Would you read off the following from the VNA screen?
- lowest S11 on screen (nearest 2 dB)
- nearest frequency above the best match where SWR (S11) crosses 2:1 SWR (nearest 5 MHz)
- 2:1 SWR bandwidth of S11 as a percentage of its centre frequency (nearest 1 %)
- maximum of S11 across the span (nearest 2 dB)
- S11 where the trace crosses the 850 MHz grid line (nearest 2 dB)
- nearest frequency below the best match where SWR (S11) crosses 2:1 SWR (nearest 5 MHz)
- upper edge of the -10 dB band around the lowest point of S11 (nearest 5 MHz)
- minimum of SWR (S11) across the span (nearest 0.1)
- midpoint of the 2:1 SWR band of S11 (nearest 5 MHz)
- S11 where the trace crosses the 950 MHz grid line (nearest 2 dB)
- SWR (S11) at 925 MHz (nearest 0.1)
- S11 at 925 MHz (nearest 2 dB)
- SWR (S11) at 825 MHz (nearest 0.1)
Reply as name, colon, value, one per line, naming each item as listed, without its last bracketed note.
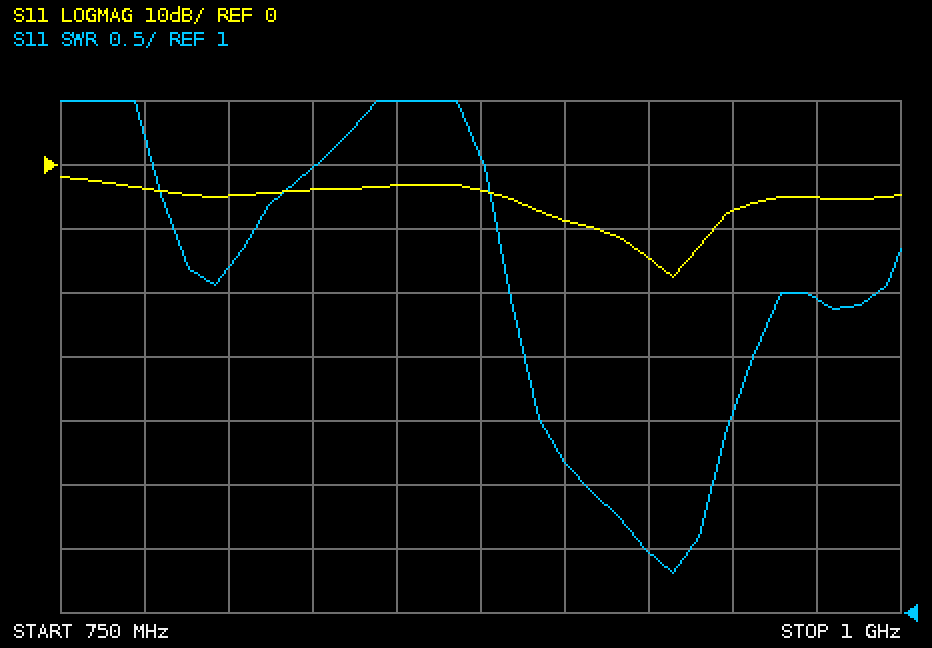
lowest S11 on screen: -18 dB
nearest frequency above the best match where SWR (S11) crosses 2:1 SWR: 945 MHz
2:1 SWR bandwidth of S11 as a percentage of its centre frequency: 4 %
maximum of S11 across the span: -2 dB
S11 where the trace crosses the 850 MHz grid line: -4 dB
nearest frequency below the best match where SWR (S11) crosses 2:1 SWR: 905 MHz
upper edge of the -10 dB band around the lowest point of S11: 945 MHz
minimum of SWR (S11) across the span: 1.3
midpoint of the 2:1 SWR band of S11: 925 MHz
S11 where the trace crosses the 950 MHz grid line: -8 dB
SWR (S11) at 925 MHz: 1.5
S11 at 925 MHz: -14 dB
SWR (S11) at 825 MHz: 4.5
